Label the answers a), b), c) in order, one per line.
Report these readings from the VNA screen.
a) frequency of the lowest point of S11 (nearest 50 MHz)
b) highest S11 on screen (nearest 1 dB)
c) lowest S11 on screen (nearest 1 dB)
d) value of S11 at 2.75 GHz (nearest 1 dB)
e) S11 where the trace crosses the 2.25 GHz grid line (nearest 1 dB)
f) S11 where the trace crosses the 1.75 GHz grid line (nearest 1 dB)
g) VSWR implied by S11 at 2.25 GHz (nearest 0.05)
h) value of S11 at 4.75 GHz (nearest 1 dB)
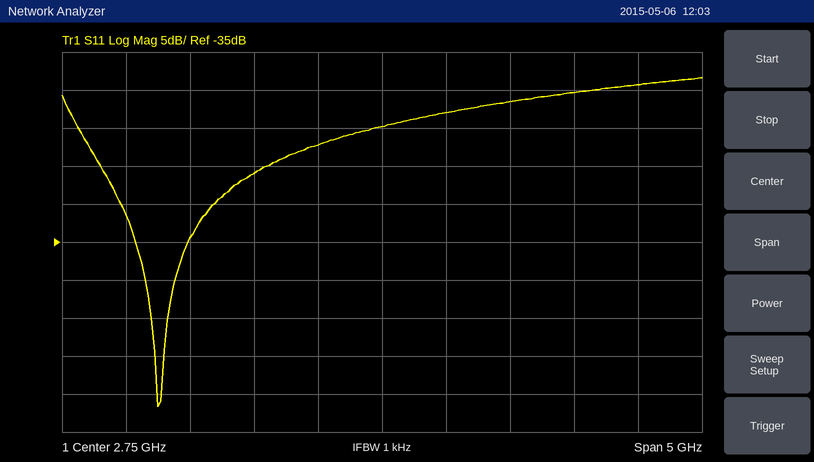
a) 1.00 GHz
b) -13 dB
c) -57 dB
d) -20 dB
e) -22 dB
f) -26 dB
g) 1.15
h) -14 dB
